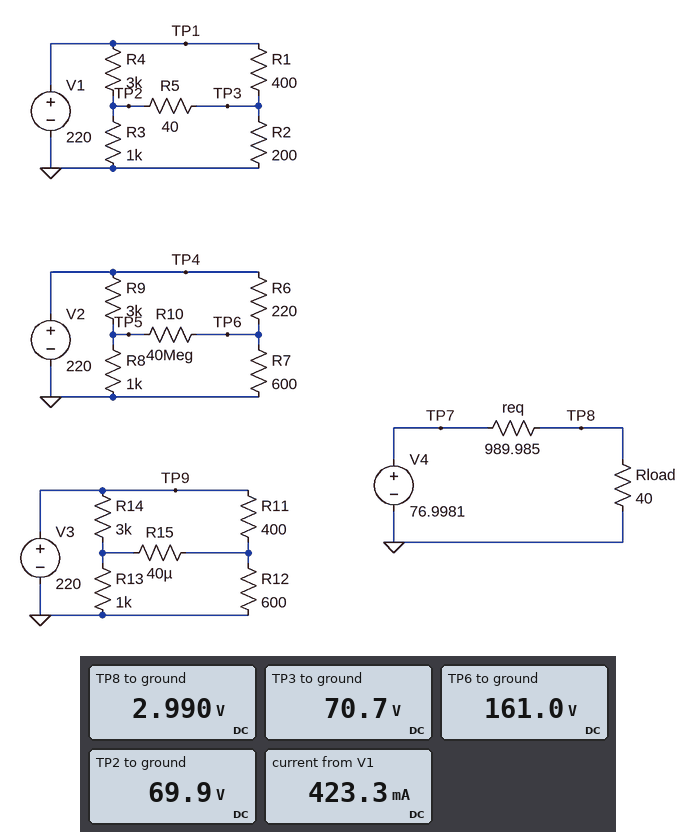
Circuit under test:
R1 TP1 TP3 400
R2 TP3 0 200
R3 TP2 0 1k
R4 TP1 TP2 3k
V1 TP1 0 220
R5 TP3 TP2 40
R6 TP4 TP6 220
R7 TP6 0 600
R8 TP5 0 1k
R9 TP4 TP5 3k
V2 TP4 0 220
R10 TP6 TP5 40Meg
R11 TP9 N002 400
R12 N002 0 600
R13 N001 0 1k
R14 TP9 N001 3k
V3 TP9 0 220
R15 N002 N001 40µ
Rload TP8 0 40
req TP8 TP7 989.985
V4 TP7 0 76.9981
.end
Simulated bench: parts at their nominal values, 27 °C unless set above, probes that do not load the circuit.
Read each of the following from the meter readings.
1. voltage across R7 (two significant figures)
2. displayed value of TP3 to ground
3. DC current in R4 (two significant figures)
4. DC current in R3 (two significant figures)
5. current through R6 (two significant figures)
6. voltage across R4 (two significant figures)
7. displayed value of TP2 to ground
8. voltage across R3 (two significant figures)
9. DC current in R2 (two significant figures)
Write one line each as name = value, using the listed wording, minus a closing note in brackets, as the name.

voltage across R7 = 160 V
displayed value of TP3 to ground = 70.7 V
DC current in R4 = 50 mA
DC current in R3 = 70 mA
current through R6 = 270 mA
voltage across R4 = 150 V
displayed value of TP2 to ground = 69.9 V
voltage across R3 = 70 V
DC current in R2 = 350 mA
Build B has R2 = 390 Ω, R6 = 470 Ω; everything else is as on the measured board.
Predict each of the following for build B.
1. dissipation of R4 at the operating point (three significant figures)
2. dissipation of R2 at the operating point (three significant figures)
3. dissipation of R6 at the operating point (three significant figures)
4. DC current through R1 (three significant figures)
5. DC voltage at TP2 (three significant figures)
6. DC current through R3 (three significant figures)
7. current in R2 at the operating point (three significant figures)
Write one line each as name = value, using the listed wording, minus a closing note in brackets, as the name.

dissipation of R4 at the operating point = 5.15 W
dissipation of R2 at the operating point = 24.6 W
dissipation of R6 at the operating point = 19.9 W
DC current through R1 = 305 mA
DC voltage at TP2 = 95.7 V
DC current through R3 = 95.7 mA
current in R2 at the operating point = 251 mA
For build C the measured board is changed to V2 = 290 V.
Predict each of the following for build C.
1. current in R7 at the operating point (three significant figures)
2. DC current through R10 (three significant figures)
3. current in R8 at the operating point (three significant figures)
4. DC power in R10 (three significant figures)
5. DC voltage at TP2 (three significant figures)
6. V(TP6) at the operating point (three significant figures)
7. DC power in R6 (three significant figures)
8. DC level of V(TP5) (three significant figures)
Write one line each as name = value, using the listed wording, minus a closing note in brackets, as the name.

current in R7 at the operating point = 354 mA
DC current through R10 = 3.49 µA
current in R8 at the operating point = 72.5 mA
DC power in R10 = 488 µW
DC voltage at TP2 = 69.9 V
V(TP6) at the operating point = 212 V
DC power in R6 = 27.5 W
DC level of V(TP5) = 72.5 V
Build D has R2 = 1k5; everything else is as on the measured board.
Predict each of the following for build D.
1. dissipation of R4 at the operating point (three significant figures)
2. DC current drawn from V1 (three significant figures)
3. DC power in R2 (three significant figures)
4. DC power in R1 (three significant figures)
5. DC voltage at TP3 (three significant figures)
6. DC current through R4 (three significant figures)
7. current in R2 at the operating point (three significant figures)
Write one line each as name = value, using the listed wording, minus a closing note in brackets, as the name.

dissipation of R4 at the operating point = 2.38 W
DC current drawn from V1 = 229 mA
DC power in R2 = 13.0 W
DC power in R1 = 16.1 W
DC voltage at TP3 = 140 V
DC current through R4 = 28.2 mA
current in R2 at the operating point = 93.2 mA
